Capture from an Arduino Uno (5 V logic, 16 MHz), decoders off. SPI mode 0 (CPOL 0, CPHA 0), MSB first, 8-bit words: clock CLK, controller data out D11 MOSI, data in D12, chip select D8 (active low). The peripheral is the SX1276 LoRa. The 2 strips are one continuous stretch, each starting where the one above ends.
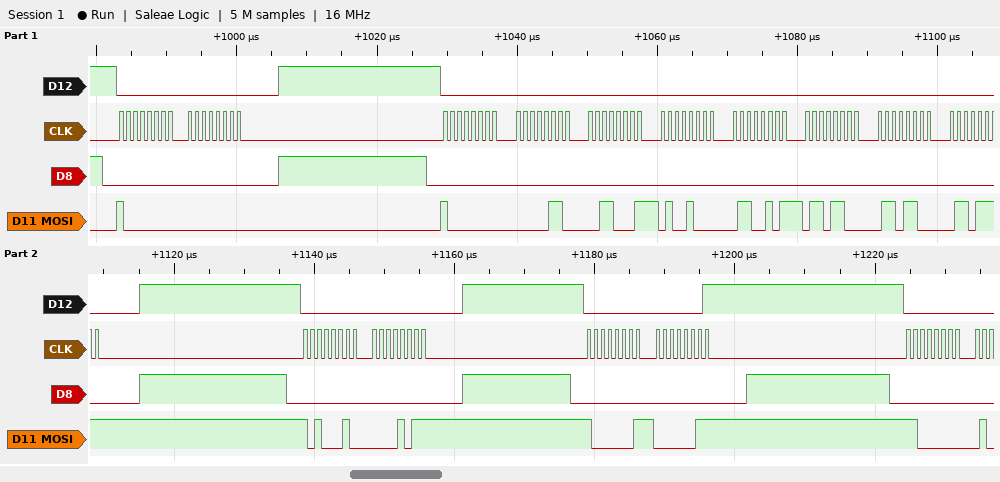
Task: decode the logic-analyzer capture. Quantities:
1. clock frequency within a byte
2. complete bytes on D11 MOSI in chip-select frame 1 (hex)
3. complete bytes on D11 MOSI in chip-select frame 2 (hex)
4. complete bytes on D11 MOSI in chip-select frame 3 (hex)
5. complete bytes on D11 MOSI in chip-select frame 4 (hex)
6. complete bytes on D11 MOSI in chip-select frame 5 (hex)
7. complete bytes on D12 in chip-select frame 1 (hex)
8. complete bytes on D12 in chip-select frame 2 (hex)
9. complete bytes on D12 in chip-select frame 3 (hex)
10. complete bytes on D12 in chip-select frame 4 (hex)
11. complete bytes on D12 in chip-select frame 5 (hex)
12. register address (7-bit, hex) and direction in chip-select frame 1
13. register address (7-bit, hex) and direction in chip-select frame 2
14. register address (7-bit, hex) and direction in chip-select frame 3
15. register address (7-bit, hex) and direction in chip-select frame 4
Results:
1 MHz
0x80 0x00
0x80 0x06 0x31 0x48 0x65 0x6C 0x6C 0x6F
0xA2 0x0B
0x81 0x03
0xC0
0x00 0x00
0x00 0x00 0x00 0x00 0x00 0x00 0x00 0x00
0x00 0x00
0x00 0x01
0x00
0x00 write
0x00 write
0x22 write
0x01 write
